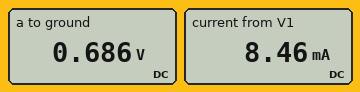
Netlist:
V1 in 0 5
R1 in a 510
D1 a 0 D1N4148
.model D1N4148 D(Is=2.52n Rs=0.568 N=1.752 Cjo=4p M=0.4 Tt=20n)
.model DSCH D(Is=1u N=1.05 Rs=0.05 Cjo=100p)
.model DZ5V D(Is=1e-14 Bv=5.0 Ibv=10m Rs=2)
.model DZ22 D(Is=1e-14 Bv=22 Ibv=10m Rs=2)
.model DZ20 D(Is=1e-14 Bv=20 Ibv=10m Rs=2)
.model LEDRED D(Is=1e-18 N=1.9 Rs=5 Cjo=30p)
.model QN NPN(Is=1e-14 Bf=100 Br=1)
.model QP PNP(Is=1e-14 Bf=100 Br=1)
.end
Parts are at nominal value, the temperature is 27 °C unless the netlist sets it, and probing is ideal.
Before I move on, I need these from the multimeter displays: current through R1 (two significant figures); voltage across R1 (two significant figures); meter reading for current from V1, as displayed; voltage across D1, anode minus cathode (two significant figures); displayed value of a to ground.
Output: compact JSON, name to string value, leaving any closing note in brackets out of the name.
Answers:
{"current through R1": "8.5 mA", "voltage across R1": "4.3 V", "meter reading for current from V1, as displayed": "8.46 mA", "voltage across D1, anode minus cathode": "690 mV", "displayed value of a to ground": "0.686 V"}
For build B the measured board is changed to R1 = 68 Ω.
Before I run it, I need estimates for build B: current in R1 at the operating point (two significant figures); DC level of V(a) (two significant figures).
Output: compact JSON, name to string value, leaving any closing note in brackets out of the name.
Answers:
{"current in R1 at the operating point": "62 mA", "DC level of V(a)": "810 mV"}
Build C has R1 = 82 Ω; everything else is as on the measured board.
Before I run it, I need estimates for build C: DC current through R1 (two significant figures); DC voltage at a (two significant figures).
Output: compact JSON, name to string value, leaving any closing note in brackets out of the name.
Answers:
{"DC current through R1": "51 mA", "DC voltage at a": "790 mV"}
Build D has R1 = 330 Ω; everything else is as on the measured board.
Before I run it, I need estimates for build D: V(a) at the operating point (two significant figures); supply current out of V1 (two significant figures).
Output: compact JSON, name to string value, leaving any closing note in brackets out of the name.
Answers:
{"V(a) at the operating point": "710 mV", "supply current out of V1": "13 mA"}
